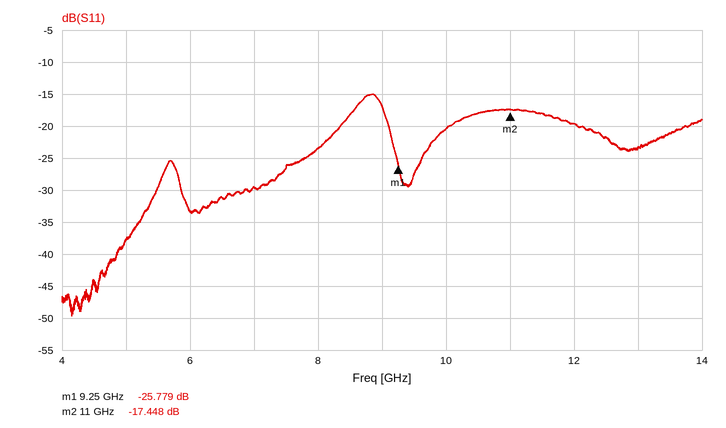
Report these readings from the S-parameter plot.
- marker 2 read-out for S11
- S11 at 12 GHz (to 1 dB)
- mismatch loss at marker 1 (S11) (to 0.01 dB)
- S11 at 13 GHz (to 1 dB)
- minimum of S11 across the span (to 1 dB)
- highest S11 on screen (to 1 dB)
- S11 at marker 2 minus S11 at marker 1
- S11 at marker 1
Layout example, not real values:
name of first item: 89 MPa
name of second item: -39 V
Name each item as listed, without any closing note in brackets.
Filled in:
marker 2 read-out for S11: -17.448 dB
S11 at 12 GHz: -20 dB
mismatch loss at marker 1 (S11): 0.01 dB
S11 at 13 GHz: -23 dB
minimum of S11 across the span: -50 dB
highest S11 on screen: -15 dB
S11 at marker 2 minus S11 at marker 1: 8.331 dB
S11 at marker 1: -25.779 dB
